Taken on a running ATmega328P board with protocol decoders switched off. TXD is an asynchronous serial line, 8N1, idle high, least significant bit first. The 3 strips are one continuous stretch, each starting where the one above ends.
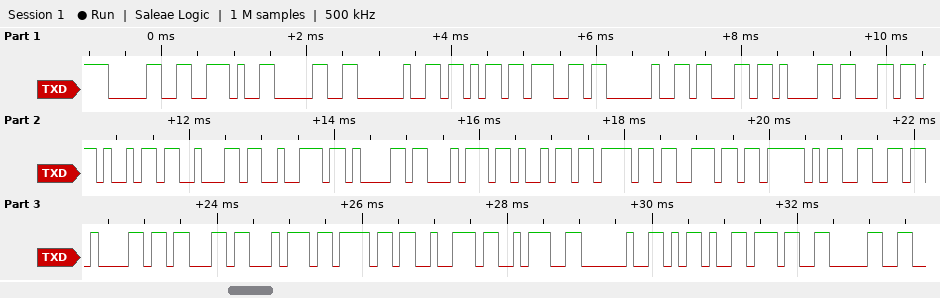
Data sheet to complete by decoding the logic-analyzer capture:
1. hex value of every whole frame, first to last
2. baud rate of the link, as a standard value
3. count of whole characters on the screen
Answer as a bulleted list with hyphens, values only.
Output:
- 30 2E 30 20 6B 67 20 63 61 6C 69 62 72 61 74 69 6F 6E 5F 66 61 63 74 6F 72 3A 20 2D 37 30
- 9600 baud
- 30
